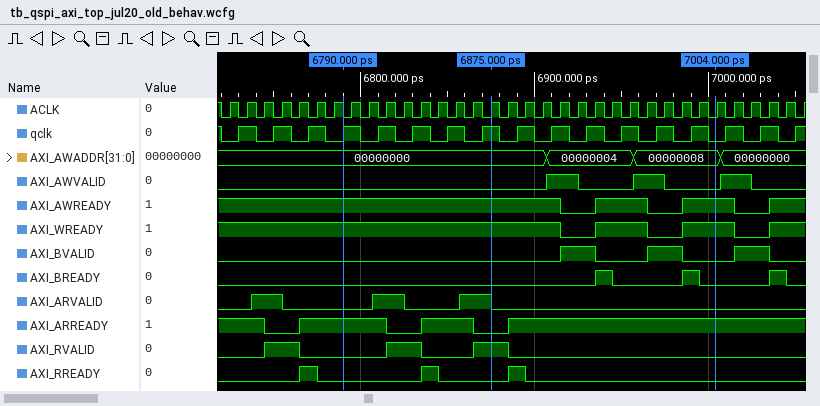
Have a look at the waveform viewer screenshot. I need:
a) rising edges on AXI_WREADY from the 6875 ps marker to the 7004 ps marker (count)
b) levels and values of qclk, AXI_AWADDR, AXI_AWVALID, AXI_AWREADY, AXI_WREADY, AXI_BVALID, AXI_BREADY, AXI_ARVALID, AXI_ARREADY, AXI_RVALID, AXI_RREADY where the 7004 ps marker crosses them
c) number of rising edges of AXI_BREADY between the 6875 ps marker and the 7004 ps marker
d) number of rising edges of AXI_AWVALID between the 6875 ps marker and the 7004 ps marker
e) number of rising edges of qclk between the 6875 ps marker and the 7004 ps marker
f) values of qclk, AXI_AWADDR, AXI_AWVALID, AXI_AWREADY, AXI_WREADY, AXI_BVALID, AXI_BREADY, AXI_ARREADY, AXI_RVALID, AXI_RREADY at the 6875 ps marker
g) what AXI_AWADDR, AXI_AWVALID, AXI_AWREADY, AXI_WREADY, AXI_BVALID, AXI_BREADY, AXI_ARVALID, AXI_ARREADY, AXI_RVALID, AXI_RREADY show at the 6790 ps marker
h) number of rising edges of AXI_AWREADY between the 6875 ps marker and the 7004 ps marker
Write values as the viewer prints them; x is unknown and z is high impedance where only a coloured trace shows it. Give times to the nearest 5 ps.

2
qclk=0, AXI_AWADDR=00000008, AXI_AWVALID=0, AXI_AWREADY=1, AXI_WREADY=1, AXI_BVALID=0, AXI_BREADY=0, AXI_ARVALID=0, AXI_ARREADY=1, AXI_RVALID=0, AXI_RREADY=0
2
2
6
qclk=1, AXI_AWADDR=00000000, AXI_AWVALID=0, AXI_AWREADY=1, AXI_WREADY=1, AXI_BVALID=0, AXI_BREADY=0, AXI_ARREADY=0, AXI_RVALID=1, AXI_RREADY=0
AXI_AWADDR=00000000, AXI_AWVALID=0, AXI_AWREADY=1, AXI_WREADY=1, AXI_BVALID=0, AXI_BREADY=0, AXI_ARVALID=0, AXI_ARREADY=1, AXI_RVALID=0, AXI_RREADY=0
2
